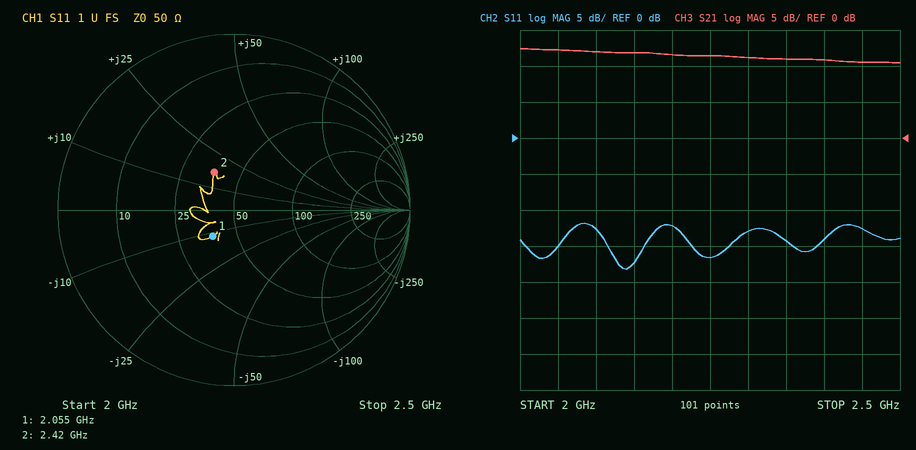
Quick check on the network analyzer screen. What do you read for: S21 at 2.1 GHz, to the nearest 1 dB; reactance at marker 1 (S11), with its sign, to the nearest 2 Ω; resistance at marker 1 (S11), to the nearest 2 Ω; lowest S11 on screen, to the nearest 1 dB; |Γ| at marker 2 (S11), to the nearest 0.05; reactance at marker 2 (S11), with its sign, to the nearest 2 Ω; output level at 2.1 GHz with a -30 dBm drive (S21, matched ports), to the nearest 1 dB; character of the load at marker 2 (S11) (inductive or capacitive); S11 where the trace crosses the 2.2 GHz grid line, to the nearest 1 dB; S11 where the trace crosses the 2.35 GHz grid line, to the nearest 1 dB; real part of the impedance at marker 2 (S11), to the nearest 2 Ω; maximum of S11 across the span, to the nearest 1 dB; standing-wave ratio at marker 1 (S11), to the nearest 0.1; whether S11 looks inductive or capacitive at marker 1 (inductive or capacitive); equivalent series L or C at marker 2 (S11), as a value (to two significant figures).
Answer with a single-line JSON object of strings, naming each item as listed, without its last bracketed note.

{"S21 at 2.1 GHz, to the nearest 1 dB": "12 dB", "reactance at marker 1 (S11), with its sign, to the nearest 2 Ω": "-12 Ω", "resistance at marker 1 (S11), to the nearest 2 Ω": "38 Ω", "lowest S11 on screen, to the nearest 1 dB": "-18 dB", "|Γ| at marker 2 (S11), to the nearest 0.05": "0.25", "reactance at marker 2 (S11), with its sign, to the nearest 2 Ω": "+16 Ω", "output level at 2.1 GHz with a -30 dBm drive (S21, matched ports), to the nearest 1 dB": "-18 dBm", "character of the load at marker 2 (S11)": "inductive", "S11 where the trace crosses the 2.2 GHz grid line, to the nearest 1 dB": "-12 dB", "S11 where the trace crosses the 2.35 GHz grid line, to the nearest 1 dB": "-14 dB", "real part of the impedance at marker 2 (S11), to the nearest 2 Ω": "36 Ω", "maximum of S11 across the span, to the nearest 1 dB": "-12 dB", "standing-wave ratio at marker 1 (S11), to the nearest 0.1": "1.5", "whether S11 looks inductive or capacitive at marker 1": "capacitive", "equivalent series L or C at marker 2 (S11), as a value": "1.1 nH"}
